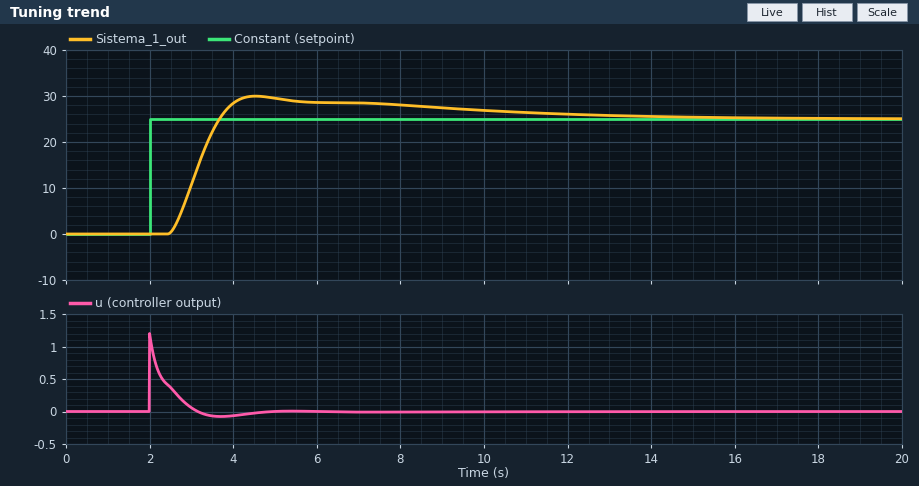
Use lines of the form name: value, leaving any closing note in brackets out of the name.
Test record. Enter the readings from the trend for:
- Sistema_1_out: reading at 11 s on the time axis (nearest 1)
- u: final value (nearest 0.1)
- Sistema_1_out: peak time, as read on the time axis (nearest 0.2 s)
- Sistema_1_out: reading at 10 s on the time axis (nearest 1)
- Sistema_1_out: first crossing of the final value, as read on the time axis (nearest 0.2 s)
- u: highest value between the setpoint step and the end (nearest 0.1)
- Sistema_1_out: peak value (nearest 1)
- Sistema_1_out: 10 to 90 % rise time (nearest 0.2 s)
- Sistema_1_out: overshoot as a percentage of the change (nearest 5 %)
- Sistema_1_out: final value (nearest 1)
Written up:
Sistema_1_out: reading at 11 s on the time axis: 26
u: final value: 0.0
Sistema_1_out: peak time, as read on the time axis: 4.6 s
Sistema_1_out: reading at 10 s on the time axis: 27
Sistema_1_out: first crossing of the final value, as read on the time axis: 3.6 s
u: highest value between the setpoint step and the end: 1.2
Sistema_1_out: peak value: 30
Sistema_1_out: 10 to 90 % rise time: 0.8 s
Sistema_1_out: overshoot as a percentage of the change: 20 %
Sistema_1_out: final value: 25
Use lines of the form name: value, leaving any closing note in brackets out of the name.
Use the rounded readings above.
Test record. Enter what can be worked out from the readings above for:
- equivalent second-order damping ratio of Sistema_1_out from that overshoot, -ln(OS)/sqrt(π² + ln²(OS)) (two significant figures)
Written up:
equivalent second-order damping ratio of Sistema_1_out from that overshoot, -ln(OS)/sqrt(π² + ln²(OS)): 0.46
